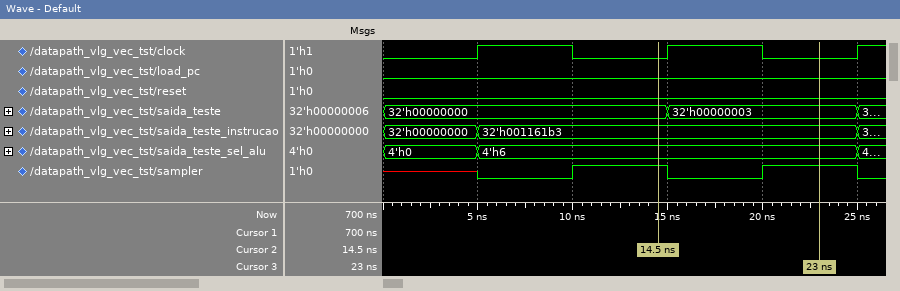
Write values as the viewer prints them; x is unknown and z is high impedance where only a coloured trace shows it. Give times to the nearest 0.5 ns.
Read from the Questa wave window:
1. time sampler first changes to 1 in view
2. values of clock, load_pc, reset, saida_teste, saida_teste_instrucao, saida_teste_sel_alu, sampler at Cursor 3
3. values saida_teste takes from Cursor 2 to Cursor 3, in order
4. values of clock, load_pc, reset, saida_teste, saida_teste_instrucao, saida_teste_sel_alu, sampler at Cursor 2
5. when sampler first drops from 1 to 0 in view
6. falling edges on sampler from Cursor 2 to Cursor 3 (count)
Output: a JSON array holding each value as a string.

["10 ns", "clock=0, load_pc=0, reset=0, saida_teste=32'h00000003, saida_teste_instrucao=32'h001161b3, saida_teste_sel_alu=4'h6, sampler=1", "32'h00000000, 32'h00000003", "clock=0, load_pc=0, reset=0, saida_teste=32'h00000000, saida_teste_instrucao=32'h001161b3, saida_teste_sel_alu=4'h6, sampler=1", "15 ns", "1"]
